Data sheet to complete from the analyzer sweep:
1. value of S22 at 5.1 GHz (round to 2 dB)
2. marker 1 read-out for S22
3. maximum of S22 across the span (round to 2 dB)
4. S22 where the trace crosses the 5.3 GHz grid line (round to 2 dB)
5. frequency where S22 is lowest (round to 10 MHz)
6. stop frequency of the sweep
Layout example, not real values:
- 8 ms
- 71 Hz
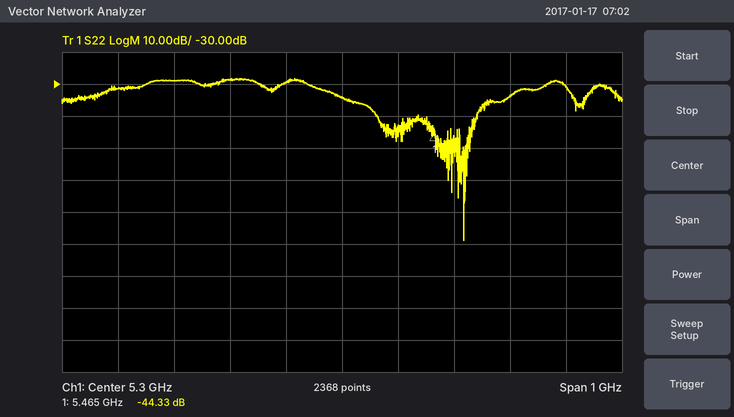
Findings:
- -28 dB
- -44.33 dB
- -28 dB
- -34 dB
- 5.52 GHz
- 5.8 GHz
